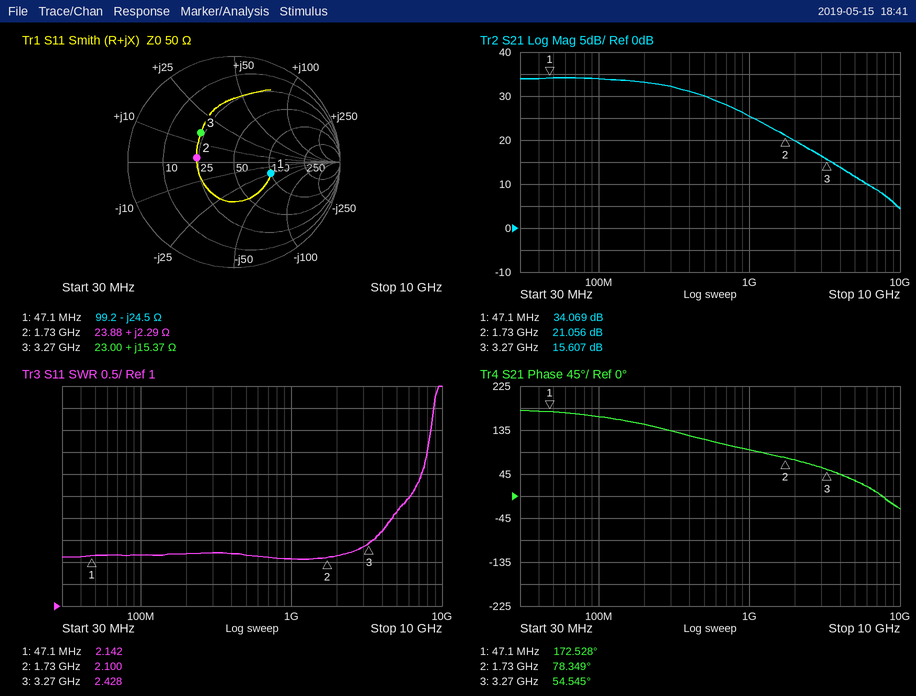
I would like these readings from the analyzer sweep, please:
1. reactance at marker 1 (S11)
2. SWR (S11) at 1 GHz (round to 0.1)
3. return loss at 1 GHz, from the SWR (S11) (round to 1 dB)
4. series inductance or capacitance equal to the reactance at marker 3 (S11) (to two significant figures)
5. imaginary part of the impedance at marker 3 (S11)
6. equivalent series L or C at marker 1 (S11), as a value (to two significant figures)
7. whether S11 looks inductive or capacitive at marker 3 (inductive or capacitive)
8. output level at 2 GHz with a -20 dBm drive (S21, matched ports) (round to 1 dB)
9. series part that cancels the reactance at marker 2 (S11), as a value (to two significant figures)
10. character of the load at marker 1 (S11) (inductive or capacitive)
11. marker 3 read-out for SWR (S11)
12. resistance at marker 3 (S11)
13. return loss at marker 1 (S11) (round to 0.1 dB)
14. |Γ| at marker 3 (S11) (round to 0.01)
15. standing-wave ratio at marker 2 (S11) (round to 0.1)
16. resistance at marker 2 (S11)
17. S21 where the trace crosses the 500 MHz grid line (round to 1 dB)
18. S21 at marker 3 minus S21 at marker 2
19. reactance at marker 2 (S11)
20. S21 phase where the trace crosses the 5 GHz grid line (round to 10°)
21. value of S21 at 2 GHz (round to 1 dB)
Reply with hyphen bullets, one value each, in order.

- -24.5 Ω
- 2.1
- 9 dB
- 750 pH
- +15.37 Ω
- 140 pF
- inductive
- 0 dBm
- 40 pF
- capacitive
- 2.428
- 23.00 Ω
- 8.8 dB
- 0.42
- 2.1
- 23.88 Ω
- 30 dB
- -5.449 dB
- +2.29 Ω
- 30°
- 20 dB
